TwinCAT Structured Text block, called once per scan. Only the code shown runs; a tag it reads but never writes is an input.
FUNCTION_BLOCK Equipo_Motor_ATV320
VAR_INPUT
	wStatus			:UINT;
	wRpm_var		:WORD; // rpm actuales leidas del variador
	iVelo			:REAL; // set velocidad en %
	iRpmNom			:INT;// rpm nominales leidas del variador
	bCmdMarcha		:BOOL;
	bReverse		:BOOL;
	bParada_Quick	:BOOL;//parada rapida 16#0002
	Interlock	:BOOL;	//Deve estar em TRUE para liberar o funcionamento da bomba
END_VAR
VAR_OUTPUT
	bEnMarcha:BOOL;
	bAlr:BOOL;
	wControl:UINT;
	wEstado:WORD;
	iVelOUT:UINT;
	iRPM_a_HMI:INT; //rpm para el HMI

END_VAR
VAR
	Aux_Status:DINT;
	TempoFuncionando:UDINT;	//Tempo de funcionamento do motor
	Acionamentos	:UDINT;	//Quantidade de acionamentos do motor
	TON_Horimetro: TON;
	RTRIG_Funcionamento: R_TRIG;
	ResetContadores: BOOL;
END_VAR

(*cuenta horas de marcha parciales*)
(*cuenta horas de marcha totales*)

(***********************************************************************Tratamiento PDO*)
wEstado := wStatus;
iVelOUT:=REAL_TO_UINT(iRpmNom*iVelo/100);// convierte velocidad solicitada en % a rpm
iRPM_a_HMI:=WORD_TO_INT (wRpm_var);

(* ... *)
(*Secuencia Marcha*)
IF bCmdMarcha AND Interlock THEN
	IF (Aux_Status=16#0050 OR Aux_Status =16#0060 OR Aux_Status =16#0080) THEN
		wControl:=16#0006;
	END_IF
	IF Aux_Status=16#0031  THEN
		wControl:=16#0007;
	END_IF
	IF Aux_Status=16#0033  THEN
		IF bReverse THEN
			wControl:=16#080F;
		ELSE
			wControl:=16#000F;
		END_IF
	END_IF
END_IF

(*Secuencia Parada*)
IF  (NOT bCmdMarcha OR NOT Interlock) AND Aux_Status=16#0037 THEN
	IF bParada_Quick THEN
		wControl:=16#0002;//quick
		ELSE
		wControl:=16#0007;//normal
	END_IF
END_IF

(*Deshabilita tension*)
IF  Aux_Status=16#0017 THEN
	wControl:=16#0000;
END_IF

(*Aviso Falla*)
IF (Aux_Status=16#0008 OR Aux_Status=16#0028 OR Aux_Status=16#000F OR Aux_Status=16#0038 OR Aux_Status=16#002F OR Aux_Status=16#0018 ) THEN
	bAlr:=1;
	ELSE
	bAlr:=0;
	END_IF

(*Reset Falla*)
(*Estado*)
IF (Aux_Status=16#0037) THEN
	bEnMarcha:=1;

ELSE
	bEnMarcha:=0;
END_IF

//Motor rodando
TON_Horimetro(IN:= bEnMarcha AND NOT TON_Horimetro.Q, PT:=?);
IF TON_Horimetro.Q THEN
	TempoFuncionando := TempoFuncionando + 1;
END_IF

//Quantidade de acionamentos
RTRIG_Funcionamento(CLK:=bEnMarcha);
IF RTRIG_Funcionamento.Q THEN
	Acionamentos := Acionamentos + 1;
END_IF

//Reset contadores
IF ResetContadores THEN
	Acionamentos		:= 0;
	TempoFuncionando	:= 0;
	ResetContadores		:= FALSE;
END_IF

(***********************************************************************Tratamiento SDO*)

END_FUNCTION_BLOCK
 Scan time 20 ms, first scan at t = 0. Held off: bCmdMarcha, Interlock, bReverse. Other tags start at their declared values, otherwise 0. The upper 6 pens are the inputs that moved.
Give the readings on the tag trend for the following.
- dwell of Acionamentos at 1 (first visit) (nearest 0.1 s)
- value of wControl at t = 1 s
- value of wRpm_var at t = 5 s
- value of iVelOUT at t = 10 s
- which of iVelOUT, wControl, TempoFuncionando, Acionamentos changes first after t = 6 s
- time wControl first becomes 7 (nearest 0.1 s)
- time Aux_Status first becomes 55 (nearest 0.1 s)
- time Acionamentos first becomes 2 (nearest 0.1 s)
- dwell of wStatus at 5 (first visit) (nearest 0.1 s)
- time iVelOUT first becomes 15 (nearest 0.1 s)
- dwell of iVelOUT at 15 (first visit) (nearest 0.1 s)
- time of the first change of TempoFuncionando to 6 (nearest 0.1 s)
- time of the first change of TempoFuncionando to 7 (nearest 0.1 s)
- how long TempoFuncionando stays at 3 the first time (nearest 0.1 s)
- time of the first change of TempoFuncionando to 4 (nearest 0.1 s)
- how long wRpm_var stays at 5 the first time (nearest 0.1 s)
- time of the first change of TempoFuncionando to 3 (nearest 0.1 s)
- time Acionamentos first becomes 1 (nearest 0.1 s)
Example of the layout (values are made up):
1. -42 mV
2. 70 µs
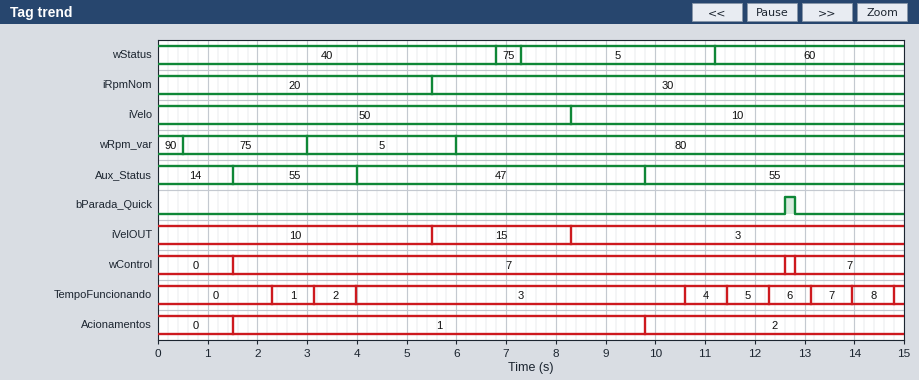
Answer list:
1. 8.3 s
2. 0
3. 5
4. 3
5. iVelOUT
6. 1.5 s
7. 1.5 s
8. 9.8 s
9. 3.9 s
10. 5.5 s
11. 2.8 s
12. 12.3 s
13. 13.1 s
14. 6.6 s
15. 10.6 s
16. 3.0 s
17. 4.0 s
18. 1.5 s
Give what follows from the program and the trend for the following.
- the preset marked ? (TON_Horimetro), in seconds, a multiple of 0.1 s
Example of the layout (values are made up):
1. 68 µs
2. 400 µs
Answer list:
1. 0.8 s
